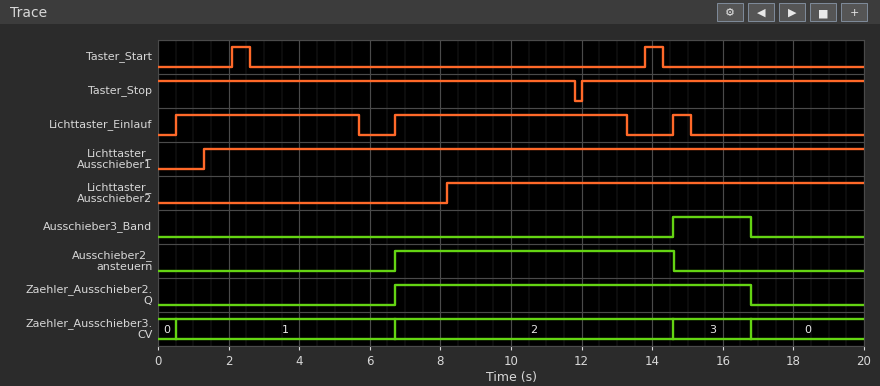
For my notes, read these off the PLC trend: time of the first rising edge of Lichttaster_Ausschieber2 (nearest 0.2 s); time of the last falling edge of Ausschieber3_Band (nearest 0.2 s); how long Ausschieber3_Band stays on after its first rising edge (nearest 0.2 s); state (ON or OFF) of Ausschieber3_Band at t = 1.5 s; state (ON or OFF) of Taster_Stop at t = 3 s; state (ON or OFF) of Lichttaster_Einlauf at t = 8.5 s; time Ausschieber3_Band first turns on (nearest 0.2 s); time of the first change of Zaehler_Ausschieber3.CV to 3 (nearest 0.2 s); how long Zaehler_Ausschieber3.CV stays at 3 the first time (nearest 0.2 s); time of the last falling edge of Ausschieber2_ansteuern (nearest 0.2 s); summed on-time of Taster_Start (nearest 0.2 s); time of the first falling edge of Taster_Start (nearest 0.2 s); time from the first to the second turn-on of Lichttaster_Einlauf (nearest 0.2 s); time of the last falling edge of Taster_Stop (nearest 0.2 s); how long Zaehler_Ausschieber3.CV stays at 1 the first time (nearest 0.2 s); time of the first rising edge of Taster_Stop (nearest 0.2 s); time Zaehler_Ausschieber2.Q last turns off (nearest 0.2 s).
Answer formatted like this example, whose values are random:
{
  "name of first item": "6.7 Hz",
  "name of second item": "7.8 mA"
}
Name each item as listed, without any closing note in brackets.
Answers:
{
  "time of the first rising edge of Lichttaster_Ausschieber2": "8.2 s",
  "time of the last falling edge of Ausschieber3_Band": "16.8 s",
  "how long Ausschieber3_Band stays on after its first rising edge": "2.2 s",
  "state (ON or OFF) of Ausschieber3_Band at t = 1.5 s": "OFF",
  "state (ON or OFF) of Taster_Stop at t = 3 s": "ON",
  "state (ON or OFF) of Lichttaster_Einlauf at t = 8.5 s": "ON",
  "time Ausschieber3_Band first turns on": "14.6 s",
  "time of the first change of Zaehler_Ausschieber3.CV to 3": "14.6 s",
  "how long Zaehler_Ausschieber3.CV stays at 3 the first time": "2.2 s",
  "time of the last falling edge of Ausschieber2_ansteuern": "14.6 s",
  "summed on-time of Taster_Start": "1.0 s",
  "time of the first falling edge of Taster_Start": "2.6 s",
  "time from the first to the second turn-on of Lichttaster_Einlauf": "6.2 s",
  "time of the last falling edge of Taster_Stop": "11.8 s",
  "how long Zaehler_Ausschieber3.CV stays at 1 the first time": "6.2 s",
  "time of the first rising edge of Taster_Stop": "12.0 s",
  "time Zaehler_Ausschieber2.Q last turns off": "16.8 s"
}
